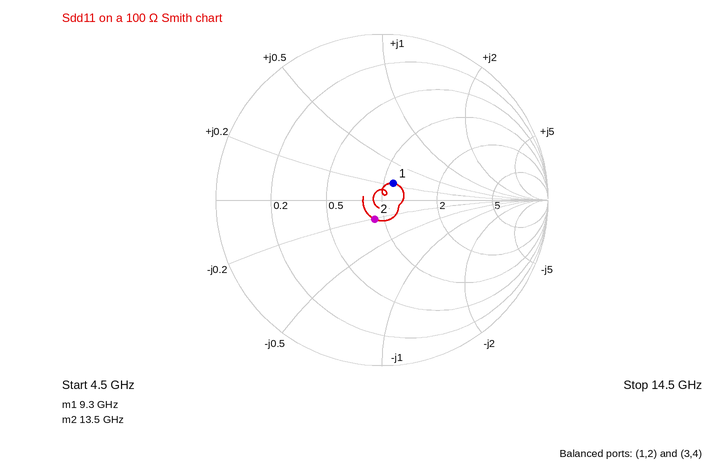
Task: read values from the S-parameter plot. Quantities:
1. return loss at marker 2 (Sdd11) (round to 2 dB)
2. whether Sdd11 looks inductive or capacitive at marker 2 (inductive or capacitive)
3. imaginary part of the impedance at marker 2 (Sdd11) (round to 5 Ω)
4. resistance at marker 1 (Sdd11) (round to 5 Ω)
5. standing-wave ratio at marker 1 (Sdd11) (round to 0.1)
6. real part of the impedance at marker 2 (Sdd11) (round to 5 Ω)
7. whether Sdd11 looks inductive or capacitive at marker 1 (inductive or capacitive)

18 dB
capacitive
-20 Ω
110 Ω
1.3
90 Ω
inductive
